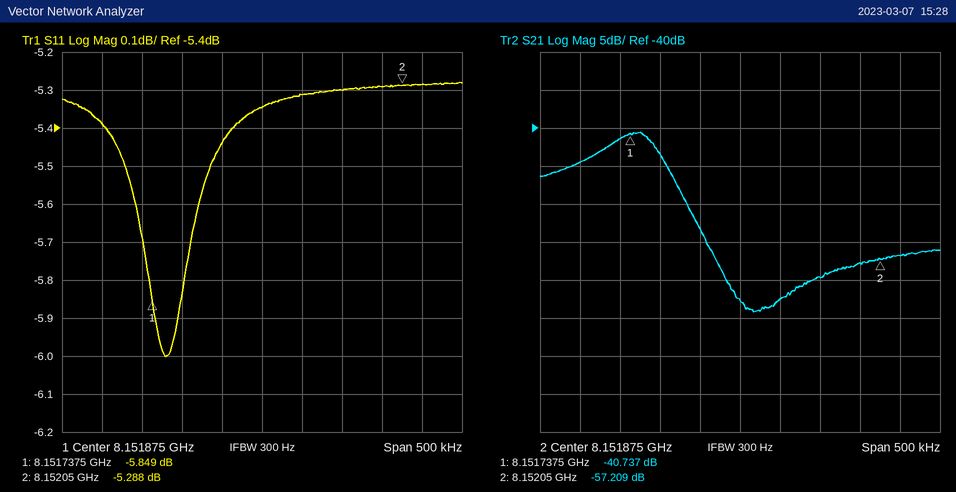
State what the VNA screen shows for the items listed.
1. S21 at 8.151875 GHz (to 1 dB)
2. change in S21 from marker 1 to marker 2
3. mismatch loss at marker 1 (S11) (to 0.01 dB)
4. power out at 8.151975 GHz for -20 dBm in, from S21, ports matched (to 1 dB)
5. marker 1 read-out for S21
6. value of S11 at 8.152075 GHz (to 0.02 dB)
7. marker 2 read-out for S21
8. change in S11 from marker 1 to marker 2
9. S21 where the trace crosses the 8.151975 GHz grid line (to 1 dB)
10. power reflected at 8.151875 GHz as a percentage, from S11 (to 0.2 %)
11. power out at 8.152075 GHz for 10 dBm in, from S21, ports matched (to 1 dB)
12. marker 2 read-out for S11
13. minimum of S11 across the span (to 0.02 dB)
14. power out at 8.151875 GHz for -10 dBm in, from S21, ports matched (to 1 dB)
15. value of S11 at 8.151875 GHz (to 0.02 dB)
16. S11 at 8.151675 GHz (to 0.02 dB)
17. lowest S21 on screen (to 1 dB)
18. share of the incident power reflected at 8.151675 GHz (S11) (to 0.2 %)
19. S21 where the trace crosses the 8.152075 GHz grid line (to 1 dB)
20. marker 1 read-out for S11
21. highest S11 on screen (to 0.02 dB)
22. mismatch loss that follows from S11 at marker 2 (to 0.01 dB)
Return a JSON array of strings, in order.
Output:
["-63 dB", "-16.472 dB", "1.31 dB", "-80 dBm", "-40.737 dB", "-5.28 dB", "-57.209 dB", "0.561 dB", "-60 dB", "29.2 %", "-47 dBm", "-5.288 dB", "-6.00 dB", "-73 dBm", "-5.34 dB", "-5.38 dB", "-64 dB", "29.0 %", "-57 dB", "-5.849 dB", "-5.28 dB", "1.52 dB"]
